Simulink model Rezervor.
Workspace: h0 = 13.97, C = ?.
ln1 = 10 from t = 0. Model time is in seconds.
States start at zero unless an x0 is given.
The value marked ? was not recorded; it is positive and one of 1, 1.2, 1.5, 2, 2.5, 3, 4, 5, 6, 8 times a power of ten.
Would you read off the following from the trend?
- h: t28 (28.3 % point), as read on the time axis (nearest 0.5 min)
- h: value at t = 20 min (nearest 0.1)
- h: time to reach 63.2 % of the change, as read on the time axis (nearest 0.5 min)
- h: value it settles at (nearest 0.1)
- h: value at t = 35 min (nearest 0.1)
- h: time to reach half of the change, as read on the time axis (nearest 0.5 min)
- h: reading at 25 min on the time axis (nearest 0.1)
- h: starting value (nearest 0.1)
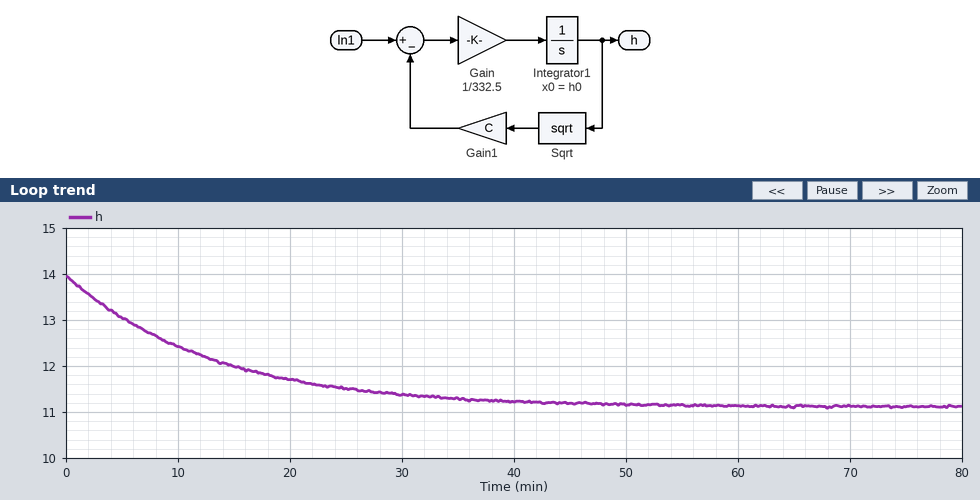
4.5 min
11.7
13.0 min
11.1
11.3
9.0 min
11.5
14.0
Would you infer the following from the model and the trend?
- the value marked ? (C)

3
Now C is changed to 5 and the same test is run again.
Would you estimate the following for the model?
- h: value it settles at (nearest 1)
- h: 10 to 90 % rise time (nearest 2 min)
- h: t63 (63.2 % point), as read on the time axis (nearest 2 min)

4
12 min
6 min
